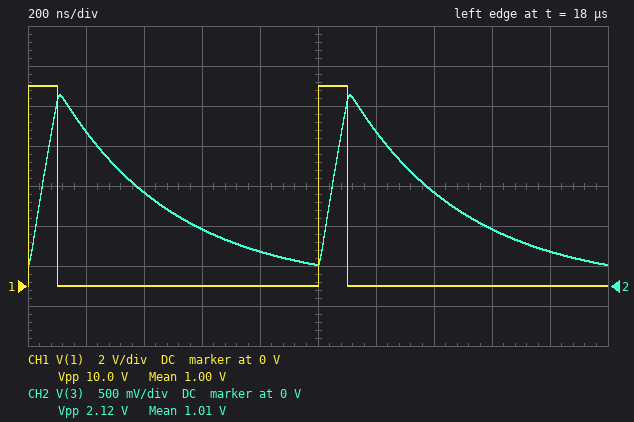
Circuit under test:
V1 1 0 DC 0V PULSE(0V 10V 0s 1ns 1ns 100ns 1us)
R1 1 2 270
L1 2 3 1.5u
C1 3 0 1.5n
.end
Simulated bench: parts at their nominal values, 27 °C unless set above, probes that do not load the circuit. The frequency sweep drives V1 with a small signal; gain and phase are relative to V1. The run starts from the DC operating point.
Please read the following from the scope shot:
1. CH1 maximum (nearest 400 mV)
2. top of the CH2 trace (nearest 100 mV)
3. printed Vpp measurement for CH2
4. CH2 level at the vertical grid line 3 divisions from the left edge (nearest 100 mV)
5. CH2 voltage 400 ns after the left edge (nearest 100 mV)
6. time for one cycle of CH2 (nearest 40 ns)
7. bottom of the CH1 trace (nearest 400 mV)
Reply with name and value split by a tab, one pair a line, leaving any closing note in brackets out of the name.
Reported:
CH1 maximum	10.0 V
top of the CH2 trace	2.4 V
printed Vpp measurement for CH2	2.12 V
CH2 level at the vertical grid line 3 divisions from the left edge	700 mV
CH2 voltage 400 ns after the left edge	1.2 V
time for one cycle of CH2	1.00 µs
bottom of the CH1 trace	0 V
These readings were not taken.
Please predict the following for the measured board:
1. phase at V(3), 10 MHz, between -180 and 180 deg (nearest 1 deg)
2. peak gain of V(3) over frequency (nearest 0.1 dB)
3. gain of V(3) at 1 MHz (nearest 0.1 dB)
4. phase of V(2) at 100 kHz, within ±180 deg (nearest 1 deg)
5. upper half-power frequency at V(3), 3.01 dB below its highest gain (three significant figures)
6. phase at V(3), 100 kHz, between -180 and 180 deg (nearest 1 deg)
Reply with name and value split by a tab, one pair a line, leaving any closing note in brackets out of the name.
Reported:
phase at V(3), 10 MHz, between -180 and 180 deg	-107 deg
peak gain of V(3) over frequency	0 dB
gain of V(3) at 1 MHz	-8.6 dB
phase of V(2) at 100 kHz, within ±180 deg	-14 deg
upper half-power frequency at V(3), 3.01 dB below its highest gain	398 kHz
phase at V(3), 100 kHz, between -180 and 180 deg	-14 deg
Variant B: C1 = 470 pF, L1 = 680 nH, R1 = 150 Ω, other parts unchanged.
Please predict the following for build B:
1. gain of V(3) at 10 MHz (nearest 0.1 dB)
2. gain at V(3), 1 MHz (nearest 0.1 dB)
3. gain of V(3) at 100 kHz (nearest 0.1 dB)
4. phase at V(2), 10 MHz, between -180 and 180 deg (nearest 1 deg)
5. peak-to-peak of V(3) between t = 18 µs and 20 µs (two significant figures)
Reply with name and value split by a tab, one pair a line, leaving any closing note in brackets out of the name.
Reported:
gain of V(3) at 10 MHz	-12.9 dB
gain at V(3), 1 MHz	-0.7 dB
gain of V(3) at 100 kHz	0 dB
phase at V(2), 10 MHz, between -180 and 180 deg	87 deg
peak-to-peak of V(3) between t = 18 µs and 20 µs	7.7 V
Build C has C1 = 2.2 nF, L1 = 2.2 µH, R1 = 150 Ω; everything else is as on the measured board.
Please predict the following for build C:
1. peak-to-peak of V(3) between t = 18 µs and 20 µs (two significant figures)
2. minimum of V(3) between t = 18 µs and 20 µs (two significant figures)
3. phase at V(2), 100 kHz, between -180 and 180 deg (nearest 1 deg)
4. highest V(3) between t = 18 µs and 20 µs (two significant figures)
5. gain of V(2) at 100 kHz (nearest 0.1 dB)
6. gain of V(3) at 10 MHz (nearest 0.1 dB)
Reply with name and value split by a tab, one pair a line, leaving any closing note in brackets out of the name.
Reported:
peak-to-peak of V(3) between t = 18 µs and 20 µs	2.5 V
minimum of V(3) between t = 18 µs and 20 µs	170 mV
phase at V(2), 100 kHz, between -180 and 180 deg	-12 deg
highest V(3) between t = 18 µs and 20 µs	2.7 V
gain of V(2) at 100 kHz	-0.2 dB
gain of V(3) at 10 MHz	-28.8 dB
